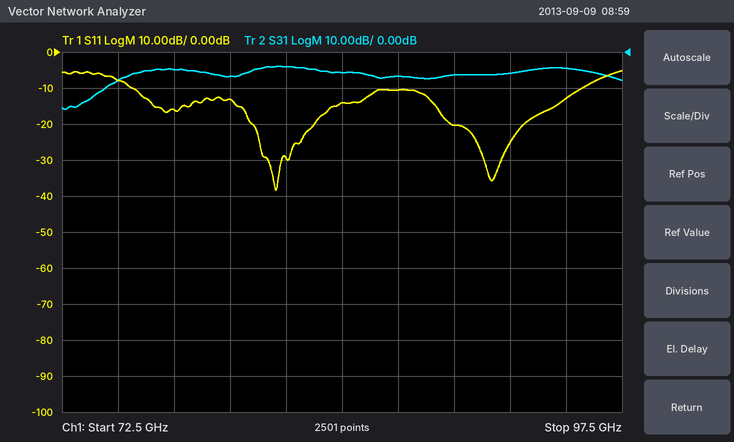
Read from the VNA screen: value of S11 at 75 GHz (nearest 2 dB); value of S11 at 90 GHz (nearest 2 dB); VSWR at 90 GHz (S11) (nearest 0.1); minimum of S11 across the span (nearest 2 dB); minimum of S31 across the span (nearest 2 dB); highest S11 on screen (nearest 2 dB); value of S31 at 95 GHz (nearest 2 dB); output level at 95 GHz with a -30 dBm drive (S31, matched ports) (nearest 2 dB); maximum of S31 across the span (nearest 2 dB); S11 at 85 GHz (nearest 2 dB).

-8 dB
-20 dB
1.2
-38 dB
-16 dB
-6 dB
-4 dB
-34 dBm
-4 dB
-14 dB
